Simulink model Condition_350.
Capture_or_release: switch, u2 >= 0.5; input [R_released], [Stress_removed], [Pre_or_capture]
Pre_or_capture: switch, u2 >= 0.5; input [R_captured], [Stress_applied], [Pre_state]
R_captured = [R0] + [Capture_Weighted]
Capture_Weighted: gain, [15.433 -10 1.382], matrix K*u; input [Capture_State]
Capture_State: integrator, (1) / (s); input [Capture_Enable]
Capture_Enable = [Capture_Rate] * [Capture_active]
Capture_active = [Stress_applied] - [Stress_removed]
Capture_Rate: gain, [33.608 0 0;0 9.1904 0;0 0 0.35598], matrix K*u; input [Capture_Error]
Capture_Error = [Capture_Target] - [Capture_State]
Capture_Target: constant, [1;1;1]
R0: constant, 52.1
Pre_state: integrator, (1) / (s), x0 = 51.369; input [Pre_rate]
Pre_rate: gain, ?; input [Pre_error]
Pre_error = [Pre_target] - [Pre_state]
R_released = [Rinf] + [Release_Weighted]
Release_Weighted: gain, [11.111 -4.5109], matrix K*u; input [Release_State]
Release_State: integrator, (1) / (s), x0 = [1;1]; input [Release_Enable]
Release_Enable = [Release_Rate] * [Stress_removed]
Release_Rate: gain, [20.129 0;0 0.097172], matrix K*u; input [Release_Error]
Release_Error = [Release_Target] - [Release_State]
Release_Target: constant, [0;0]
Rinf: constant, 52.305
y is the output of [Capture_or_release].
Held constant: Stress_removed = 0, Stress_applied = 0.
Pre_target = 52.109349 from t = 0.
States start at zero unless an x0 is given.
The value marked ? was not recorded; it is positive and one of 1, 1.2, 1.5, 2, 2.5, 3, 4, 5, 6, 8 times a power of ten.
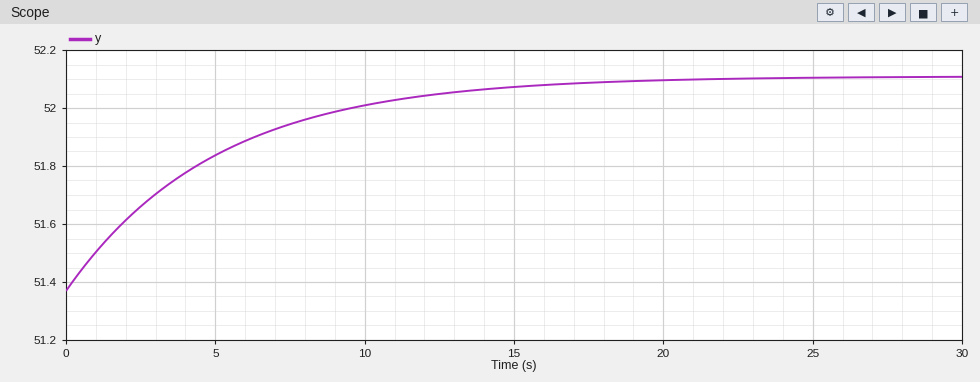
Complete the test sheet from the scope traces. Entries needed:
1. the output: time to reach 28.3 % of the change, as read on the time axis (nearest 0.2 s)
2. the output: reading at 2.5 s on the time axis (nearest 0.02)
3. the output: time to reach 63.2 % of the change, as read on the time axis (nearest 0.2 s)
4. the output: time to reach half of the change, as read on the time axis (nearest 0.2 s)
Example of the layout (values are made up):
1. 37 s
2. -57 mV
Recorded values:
1. 1.6 s
2. 51.66
3. 5.0 s
4. 3.4 s
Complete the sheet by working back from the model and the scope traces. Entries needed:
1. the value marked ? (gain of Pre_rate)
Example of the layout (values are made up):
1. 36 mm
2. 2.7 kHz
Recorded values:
1. 0.2
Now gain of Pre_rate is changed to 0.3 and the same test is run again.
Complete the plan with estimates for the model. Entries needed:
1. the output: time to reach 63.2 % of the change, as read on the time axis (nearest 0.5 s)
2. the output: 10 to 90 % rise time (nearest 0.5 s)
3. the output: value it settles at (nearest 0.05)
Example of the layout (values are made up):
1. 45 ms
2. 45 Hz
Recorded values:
1. 3.5 s
2. 7.5 s
3. 52.10
